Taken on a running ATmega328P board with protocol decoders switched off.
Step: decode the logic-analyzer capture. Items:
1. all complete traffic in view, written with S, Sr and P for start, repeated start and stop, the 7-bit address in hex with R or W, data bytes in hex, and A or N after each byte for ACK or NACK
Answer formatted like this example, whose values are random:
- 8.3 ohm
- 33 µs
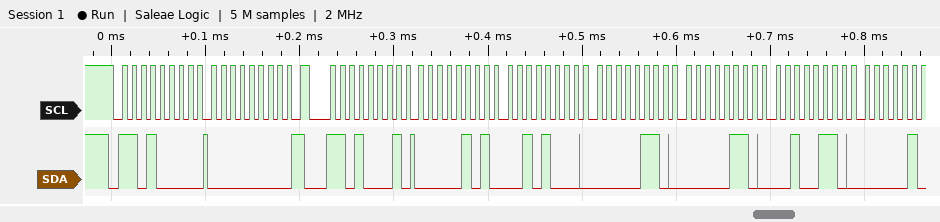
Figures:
- S 68W A 00 A Sr 68R A 05 A 28 A 06 A 06 A 26 A
